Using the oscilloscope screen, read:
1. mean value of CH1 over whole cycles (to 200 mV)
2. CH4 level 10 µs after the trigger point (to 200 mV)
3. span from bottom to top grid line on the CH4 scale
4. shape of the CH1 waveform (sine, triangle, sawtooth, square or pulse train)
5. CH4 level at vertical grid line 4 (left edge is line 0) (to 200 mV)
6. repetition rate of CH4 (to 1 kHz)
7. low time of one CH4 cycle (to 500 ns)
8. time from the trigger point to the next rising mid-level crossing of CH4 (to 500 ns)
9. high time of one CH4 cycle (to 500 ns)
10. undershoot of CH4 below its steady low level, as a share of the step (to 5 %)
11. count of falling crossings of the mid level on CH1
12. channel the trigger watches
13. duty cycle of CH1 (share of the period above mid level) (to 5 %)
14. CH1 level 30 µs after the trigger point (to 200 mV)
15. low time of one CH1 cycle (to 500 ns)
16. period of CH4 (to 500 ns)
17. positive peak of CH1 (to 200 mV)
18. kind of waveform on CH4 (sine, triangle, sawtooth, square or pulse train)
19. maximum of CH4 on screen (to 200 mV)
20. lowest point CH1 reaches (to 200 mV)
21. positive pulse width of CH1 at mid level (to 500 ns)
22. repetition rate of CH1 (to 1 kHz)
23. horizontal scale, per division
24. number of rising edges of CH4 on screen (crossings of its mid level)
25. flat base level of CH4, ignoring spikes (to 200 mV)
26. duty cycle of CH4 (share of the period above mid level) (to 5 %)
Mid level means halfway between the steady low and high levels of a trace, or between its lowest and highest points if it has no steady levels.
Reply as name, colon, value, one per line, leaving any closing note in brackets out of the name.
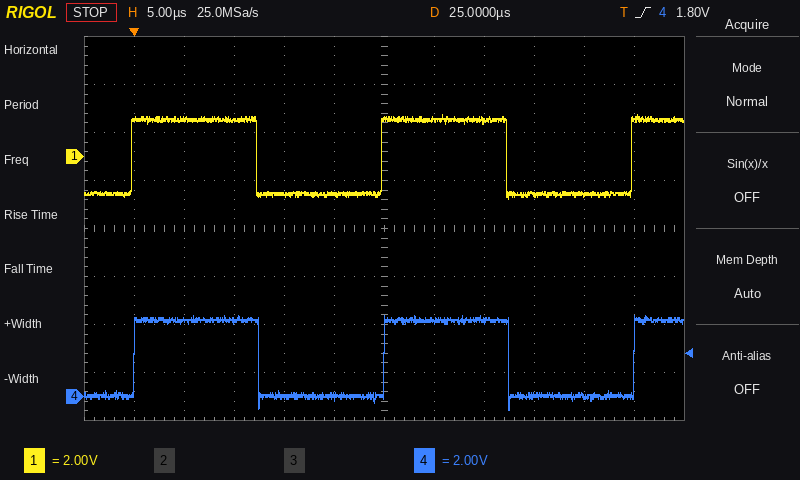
mean value of CH1 over whole cycles: 0.0 V
CH4 level 10 µs after the trigger point: 3.2 V
span from bottom to top grid line on the CH4 scale: 16 V
shape of the CH1 waveform: square
CH4 level at vertical grid line 4 (left edge is line 0): 0.0 V
repetition rate of CH4: 40 kHz
low time of one CH4 cycle: 12.5 µs
time from the trigger point to the next rising mid-level crossing of CH4: 25.0 µs
high time of one CH4 cycle: 12.5 µs
undershoot of CH4 below its steady low level, as a share of the step: 20 %
count of falling crossings of the mid level on CH1: 2
channel the trigger watches: CH4
duty cycle of CH1 (share of the period above mid level): 50 %
CH1 level 30 µs after the trigger point: 1.6 V
low time of one CH1 cycle: 12.5 µs
period of CH4: 25.0 µs
positive peak of CH1: 1.8 V
kind of waveform on CH4: square
maximum of CH4 on screen: 3.4 V
lowest point CH1 reaches: -1.8 V
positive pulse width of CH1 at mid level: 12.5 µs
repetition rate of CH1: 40 kHz
horizontal scale, per division: 5 µs
number of rising edges of CH4 on screen: 3
flat base level of CH4, ignoring spikes: 0.0 V
duty cycle of CH4 (share of the period above mid level): 50 %
